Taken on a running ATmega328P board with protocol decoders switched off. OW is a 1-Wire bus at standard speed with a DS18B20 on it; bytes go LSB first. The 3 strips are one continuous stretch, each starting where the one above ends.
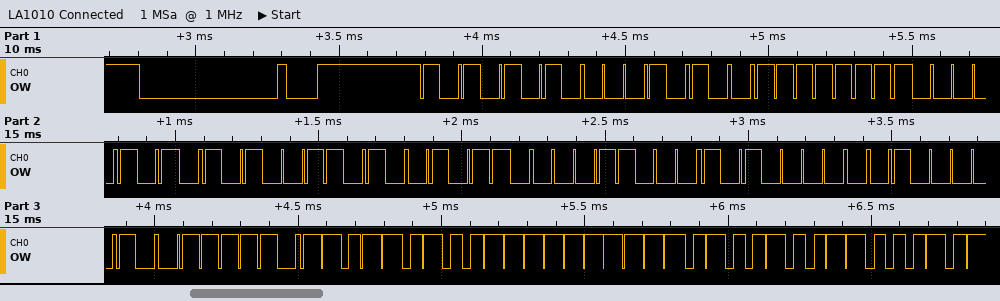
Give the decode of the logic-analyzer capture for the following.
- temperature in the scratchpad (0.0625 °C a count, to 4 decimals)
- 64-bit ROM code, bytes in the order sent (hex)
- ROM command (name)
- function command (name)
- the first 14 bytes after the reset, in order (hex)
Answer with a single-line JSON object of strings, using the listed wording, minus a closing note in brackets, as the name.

{"temperature in the scratchpad": "-13.1875 °C", "64-bit ROM code, bytes in the order sent": "28 FF 50 65 69 18 05 42", "ROM command": "Match ROM", "function command": "Read Scratchpad", "the first 14 bytes after the reset, in order": "55 28 FF 50 65 69 18 05 42 BE 2D FF 4B 46"}
